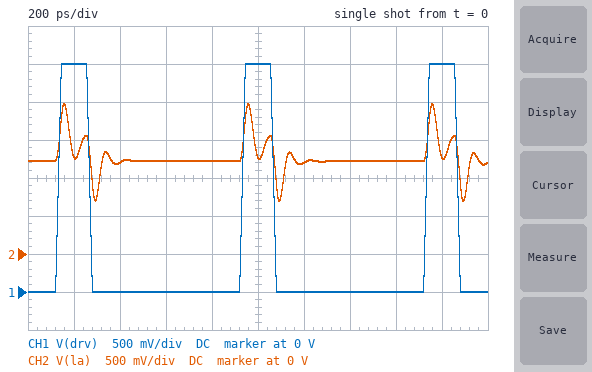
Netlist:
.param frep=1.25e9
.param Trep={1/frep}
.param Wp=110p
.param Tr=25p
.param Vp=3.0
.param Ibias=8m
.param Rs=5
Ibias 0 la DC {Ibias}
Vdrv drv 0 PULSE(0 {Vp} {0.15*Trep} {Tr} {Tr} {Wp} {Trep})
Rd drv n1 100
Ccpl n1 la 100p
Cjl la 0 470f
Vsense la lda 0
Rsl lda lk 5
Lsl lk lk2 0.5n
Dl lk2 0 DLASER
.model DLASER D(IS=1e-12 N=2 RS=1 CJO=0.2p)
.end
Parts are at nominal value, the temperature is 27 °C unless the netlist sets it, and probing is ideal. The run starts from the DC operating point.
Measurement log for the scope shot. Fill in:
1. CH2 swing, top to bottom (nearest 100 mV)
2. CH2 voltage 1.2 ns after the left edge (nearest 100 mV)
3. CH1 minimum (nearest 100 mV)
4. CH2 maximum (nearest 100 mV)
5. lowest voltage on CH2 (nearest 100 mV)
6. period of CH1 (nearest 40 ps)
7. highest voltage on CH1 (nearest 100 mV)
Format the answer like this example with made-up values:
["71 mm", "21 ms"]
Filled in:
["1.3 V", "1.2 V", "0 V", "2.0 V", "700 mV", "800 ps", "3.0 V"]
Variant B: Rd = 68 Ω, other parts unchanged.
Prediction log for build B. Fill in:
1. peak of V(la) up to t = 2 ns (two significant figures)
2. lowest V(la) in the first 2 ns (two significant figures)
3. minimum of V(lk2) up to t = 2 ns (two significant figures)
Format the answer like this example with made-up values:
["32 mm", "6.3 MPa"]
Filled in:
["2.2 V", "550 mV", "980 mV"]
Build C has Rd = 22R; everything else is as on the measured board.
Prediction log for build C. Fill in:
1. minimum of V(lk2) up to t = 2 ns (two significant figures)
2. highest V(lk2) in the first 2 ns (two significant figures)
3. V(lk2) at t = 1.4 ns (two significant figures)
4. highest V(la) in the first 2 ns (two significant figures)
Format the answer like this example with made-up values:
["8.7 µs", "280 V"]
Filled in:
["940 mV", "1.4 V", "1.1 V", "3.1 V"]
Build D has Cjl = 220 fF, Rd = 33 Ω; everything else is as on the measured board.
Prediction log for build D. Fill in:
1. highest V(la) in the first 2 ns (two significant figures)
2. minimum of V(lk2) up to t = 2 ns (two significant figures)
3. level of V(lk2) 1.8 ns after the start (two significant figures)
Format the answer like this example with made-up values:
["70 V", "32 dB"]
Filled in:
["2.9 V", "1.1 V", "1.4 V"]
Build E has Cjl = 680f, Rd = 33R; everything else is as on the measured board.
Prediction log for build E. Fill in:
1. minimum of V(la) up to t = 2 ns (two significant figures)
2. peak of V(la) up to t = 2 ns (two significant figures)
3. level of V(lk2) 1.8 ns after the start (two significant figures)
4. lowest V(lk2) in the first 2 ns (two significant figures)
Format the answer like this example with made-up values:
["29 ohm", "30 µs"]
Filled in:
["340 mV", "2.7 V", "1.4 V", "840 mV"]
